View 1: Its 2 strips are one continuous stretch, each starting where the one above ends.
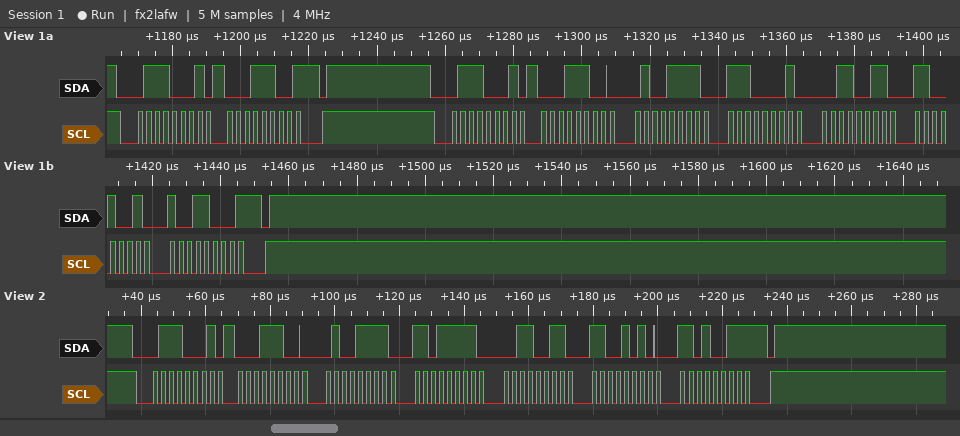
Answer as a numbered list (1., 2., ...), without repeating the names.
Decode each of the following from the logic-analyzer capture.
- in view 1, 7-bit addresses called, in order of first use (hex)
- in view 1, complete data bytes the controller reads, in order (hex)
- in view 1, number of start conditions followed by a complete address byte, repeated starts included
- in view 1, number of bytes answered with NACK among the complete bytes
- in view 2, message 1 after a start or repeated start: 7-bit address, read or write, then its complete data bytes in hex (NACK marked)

1. 0x38
2. 1C 1C 4F E1 33 C9 98
3. 2
4. 2
5. 0x38 read: 1C 4F DF 33 CA D3 NACK
